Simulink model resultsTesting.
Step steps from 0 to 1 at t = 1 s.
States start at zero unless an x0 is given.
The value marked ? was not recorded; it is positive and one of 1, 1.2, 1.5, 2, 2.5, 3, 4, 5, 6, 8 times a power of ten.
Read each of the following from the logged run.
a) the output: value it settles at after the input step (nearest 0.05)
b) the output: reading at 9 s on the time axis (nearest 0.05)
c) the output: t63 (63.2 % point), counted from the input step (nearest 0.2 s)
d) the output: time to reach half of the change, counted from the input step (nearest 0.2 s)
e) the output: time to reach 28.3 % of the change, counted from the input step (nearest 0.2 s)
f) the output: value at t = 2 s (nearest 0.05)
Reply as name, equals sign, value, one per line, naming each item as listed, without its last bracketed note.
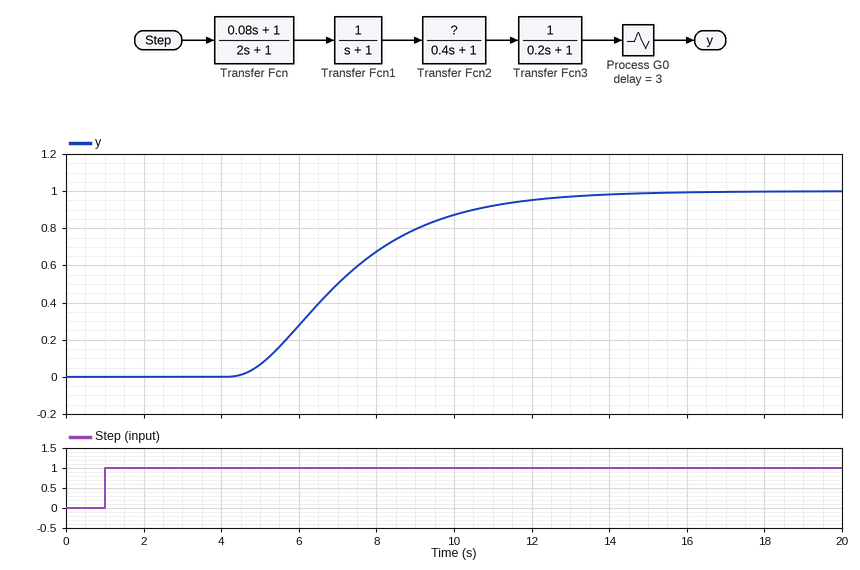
the output: value it settles at after the input step = 1.00
the output: reading at 9 s on the time axis = 0.80
the output: t63 (63.2 % point), counted from the input step = 6.8 s
the output: time to reach half of the change, counted from the input step = 6.0 s
the output: time to reach 28.3 % of the change, counted from the input step = 5.0 s
the output: value at t = 2 s = 0.00
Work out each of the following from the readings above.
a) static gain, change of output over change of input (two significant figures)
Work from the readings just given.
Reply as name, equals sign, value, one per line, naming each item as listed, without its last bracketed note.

static gain, change of output over change of input = 1.0
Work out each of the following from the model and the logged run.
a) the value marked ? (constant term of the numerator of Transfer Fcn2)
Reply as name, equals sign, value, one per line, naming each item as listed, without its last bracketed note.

the value marked ? = 1
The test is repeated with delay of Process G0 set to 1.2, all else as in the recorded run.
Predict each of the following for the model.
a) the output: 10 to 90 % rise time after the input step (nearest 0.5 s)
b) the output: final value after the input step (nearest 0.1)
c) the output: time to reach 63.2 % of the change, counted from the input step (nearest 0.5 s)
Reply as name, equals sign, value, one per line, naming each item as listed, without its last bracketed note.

the output: 10 to 90 % rise time after the input step = 5.5 s
the output: final value after the input step = 1.0
the output: time to reach 63.2 % of the change, counted from the input step = 5.0 s
